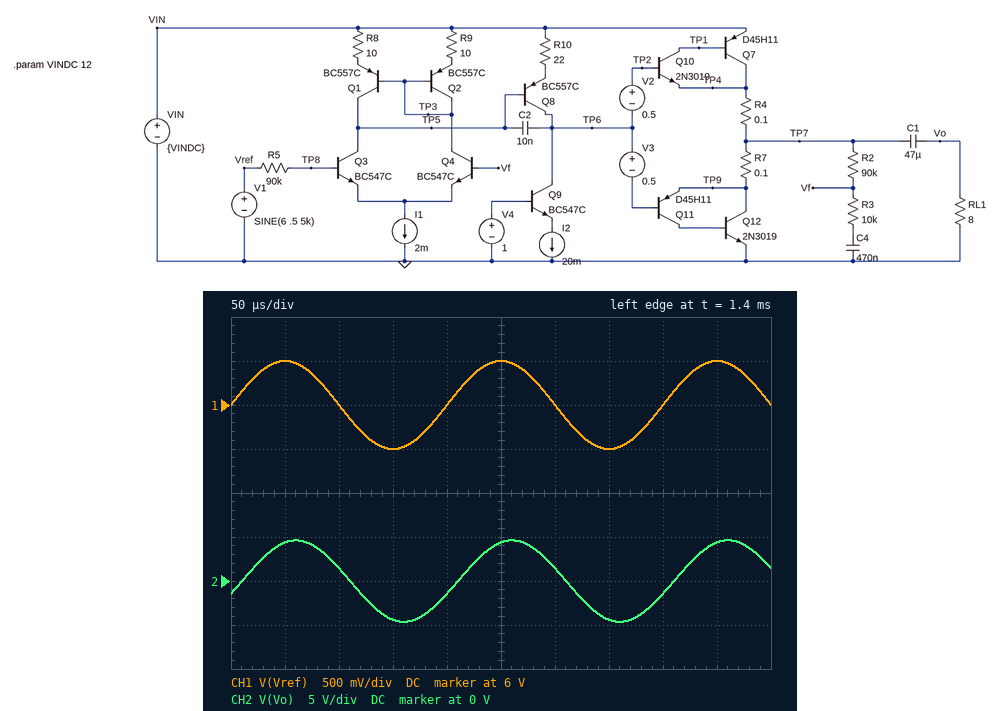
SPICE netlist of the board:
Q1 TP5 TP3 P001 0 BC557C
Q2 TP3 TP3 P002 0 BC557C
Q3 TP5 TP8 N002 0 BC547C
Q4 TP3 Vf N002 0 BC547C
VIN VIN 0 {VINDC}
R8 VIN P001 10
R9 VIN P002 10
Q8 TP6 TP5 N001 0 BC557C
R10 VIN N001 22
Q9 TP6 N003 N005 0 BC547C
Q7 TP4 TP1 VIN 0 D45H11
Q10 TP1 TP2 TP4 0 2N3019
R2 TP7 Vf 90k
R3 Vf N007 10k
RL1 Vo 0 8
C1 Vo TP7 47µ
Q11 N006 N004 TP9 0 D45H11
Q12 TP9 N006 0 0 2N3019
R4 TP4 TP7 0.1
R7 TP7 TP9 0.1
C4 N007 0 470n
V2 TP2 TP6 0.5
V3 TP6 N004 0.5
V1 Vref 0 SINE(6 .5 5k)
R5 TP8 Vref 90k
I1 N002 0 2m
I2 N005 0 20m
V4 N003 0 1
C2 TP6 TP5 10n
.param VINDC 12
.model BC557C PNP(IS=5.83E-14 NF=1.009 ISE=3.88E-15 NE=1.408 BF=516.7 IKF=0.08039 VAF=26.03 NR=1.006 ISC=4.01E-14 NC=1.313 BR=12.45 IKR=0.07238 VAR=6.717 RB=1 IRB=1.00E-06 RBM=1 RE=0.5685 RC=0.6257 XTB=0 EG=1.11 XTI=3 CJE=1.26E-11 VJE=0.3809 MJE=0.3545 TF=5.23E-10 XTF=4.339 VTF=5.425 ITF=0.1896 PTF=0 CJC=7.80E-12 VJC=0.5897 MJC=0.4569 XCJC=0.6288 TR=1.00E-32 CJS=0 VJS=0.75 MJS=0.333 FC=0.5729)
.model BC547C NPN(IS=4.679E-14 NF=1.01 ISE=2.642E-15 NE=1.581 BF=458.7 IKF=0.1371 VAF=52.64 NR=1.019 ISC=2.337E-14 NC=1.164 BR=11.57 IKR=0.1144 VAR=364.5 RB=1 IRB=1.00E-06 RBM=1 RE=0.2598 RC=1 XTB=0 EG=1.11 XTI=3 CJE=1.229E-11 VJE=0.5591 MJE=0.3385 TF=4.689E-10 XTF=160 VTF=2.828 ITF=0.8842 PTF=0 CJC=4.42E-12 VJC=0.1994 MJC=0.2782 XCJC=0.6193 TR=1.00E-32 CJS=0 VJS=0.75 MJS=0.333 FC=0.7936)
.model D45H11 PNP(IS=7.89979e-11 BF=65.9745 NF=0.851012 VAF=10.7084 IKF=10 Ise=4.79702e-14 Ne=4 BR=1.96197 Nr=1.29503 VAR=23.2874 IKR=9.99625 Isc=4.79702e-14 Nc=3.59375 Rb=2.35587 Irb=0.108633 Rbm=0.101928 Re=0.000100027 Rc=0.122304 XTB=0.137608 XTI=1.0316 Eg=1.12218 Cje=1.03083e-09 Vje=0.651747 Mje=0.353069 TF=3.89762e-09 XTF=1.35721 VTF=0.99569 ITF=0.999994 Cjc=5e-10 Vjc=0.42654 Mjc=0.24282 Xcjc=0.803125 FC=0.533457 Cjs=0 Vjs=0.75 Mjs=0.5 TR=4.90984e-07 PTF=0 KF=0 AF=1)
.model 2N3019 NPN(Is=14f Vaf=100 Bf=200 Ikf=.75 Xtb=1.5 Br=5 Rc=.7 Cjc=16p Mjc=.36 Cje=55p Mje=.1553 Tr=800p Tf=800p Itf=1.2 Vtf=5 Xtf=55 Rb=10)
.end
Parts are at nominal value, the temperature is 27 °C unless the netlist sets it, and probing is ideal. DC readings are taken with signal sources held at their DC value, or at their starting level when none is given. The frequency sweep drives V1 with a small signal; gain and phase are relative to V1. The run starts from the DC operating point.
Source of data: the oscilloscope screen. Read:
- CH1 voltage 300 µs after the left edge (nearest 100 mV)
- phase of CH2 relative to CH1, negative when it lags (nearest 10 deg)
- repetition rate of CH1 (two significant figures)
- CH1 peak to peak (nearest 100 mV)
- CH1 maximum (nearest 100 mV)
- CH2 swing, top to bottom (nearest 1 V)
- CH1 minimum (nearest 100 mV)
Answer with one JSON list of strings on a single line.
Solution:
["6.0 V", "-20 deg", "5.0 kHz", "1.0 V", "6.5 V", "9 V", "5.5 V"]
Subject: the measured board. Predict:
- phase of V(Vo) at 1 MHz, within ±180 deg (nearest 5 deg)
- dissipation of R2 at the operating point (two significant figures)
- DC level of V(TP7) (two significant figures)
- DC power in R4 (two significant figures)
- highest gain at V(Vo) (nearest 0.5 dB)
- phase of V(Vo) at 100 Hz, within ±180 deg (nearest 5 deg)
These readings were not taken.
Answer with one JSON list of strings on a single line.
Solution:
["125 deg", "340 nW", "6.0 V", "900 µW", "19.5 dB", "95 deg"]
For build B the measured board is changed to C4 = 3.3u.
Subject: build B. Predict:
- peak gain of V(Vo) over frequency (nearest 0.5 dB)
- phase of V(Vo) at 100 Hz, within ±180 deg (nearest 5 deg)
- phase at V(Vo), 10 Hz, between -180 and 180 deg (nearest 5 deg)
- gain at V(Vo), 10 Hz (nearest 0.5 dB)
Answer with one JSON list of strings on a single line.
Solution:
["19.5 dB", "80 deg", "110 deg", "-13.5 dB"]
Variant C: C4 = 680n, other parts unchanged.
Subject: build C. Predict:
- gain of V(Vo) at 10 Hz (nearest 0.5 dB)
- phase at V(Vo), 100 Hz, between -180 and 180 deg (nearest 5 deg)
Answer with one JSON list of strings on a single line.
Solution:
["-20.5 dB", "90 deg"]
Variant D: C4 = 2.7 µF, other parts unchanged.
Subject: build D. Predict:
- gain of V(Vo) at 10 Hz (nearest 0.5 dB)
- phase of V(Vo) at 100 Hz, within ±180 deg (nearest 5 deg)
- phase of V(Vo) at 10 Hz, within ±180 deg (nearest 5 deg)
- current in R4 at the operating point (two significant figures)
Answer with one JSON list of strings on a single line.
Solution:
["-14.0 dB", "80 deg", "115 deg", "95 mA"]
